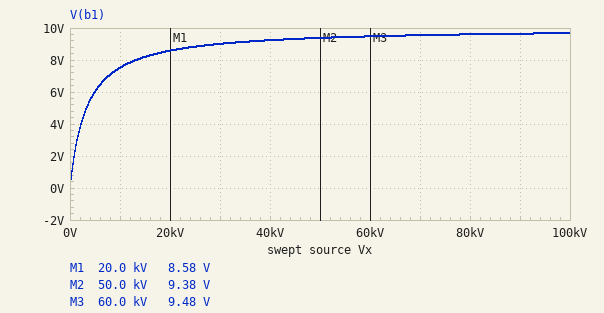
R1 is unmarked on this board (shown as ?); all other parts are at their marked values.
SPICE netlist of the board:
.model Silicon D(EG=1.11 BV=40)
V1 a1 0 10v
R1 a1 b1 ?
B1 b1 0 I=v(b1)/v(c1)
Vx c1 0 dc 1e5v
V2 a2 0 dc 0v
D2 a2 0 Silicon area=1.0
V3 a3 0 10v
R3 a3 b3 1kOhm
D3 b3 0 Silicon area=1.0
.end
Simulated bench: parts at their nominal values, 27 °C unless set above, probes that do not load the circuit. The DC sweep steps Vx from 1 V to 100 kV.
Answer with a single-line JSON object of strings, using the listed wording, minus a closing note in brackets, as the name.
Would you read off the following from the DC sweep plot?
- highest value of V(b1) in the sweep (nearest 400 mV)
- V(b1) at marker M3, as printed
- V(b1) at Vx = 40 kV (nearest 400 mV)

{"highest value of V(b1) in the sweep": "9.6 V", "V(b1) at marker M3, as printed": "9.48 V", "V(b1) at Vx = 40 kV": "9.2 V"}
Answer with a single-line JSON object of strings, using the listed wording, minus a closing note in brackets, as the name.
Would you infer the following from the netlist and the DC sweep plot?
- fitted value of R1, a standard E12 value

{"fitted value of R1, a standard E12 value": "3.3 kΩ"}
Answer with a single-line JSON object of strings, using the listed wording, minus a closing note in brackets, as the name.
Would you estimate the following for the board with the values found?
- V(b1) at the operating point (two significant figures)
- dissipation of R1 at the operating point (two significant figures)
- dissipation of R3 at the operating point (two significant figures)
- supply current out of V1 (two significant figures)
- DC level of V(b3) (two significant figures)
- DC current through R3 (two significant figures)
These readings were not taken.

{"V(b1) at the operating point": "9.7 V", "dissipation of R1 at the operating point": "31 µW", "dissipation of R3 at the operating point": "86 mW", "supply current out of V1": "97 µA", "DC level of V(b3)": "710 mV", "DC current through R3": "9.3 mA"}
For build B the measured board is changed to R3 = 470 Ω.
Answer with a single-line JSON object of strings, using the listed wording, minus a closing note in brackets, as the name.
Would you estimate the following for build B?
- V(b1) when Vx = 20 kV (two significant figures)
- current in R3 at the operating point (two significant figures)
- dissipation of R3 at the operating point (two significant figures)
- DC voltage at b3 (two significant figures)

{"V(b1) when Vx = 20 kV": "8.6 V", "current in R3 at the operating point": "20 mA", "dissipation of R3 at the operating point": "180 mW", "DC voltage at b3": "730 mV"}
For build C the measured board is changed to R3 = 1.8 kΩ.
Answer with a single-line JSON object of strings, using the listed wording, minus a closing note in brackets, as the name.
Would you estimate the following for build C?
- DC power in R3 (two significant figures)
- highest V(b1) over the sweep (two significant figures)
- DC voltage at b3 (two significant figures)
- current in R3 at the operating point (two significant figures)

{"DC power in R3": "48 mW", "highest V(b1) over the sweep": "9.7 V", "DC voltage at b3": "700 mV", "current in R3 at the operating point": "5.2 mA"}
